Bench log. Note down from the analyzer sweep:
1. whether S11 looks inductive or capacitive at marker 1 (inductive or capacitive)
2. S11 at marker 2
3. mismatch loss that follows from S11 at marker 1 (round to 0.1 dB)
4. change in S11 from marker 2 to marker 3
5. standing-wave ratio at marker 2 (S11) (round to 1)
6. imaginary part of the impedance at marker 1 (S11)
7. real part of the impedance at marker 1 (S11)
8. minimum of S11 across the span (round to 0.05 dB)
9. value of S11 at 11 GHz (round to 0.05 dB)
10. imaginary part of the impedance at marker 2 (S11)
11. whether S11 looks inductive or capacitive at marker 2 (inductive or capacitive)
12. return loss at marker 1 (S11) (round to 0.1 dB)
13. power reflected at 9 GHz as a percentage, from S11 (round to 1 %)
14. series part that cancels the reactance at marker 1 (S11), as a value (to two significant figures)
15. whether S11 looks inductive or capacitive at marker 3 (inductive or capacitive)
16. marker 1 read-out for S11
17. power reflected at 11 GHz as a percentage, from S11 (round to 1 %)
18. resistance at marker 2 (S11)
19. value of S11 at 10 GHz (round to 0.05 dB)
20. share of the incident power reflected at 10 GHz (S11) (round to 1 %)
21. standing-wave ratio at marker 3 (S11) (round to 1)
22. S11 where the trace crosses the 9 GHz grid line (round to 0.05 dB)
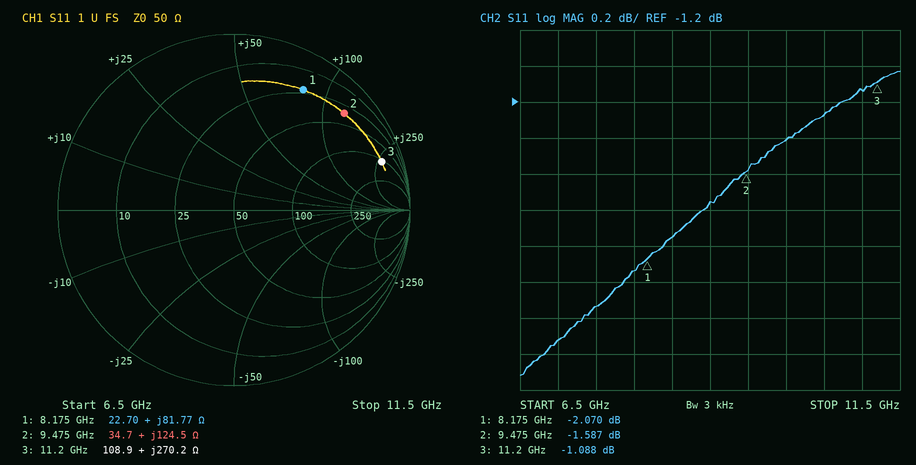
inductive
-1.587 dB
4.2 dB
0.499 dB
11
+81.77 Ω
22.70 Ω
-2.70 dB
-1.15 dB
+124.5 Ω
inductive
2.1 dB
67 %
240 fF
inductive
-2.070 dB
77 %
34.7 Ω
-1.40 dB
72 %
16
-1.75 dB
